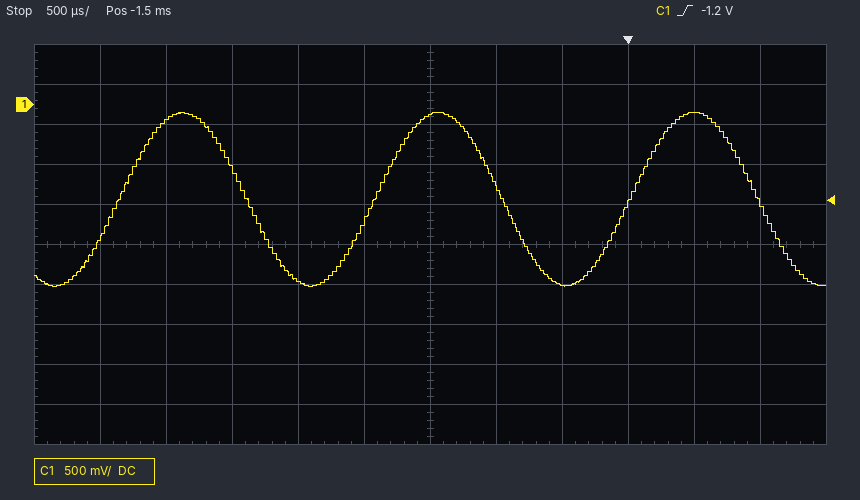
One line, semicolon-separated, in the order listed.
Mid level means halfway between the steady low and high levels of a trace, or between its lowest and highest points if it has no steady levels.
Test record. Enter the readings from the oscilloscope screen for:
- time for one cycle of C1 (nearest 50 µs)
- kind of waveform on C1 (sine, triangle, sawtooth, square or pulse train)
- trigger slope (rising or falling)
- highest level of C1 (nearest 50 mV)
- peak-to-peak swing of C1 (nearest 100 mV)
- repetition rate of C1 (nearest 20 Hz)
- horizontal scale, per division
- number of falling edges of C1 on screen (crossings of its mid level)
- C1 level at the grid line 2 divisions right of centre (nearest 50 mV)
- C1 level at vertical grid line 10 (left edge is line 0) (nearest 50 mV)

1.95 ms; sine; rising; -100 mV; 2.20 V; 520 Hz; 500 µs; 3; -2.25 V; -100 mV
